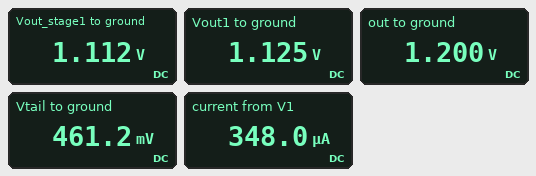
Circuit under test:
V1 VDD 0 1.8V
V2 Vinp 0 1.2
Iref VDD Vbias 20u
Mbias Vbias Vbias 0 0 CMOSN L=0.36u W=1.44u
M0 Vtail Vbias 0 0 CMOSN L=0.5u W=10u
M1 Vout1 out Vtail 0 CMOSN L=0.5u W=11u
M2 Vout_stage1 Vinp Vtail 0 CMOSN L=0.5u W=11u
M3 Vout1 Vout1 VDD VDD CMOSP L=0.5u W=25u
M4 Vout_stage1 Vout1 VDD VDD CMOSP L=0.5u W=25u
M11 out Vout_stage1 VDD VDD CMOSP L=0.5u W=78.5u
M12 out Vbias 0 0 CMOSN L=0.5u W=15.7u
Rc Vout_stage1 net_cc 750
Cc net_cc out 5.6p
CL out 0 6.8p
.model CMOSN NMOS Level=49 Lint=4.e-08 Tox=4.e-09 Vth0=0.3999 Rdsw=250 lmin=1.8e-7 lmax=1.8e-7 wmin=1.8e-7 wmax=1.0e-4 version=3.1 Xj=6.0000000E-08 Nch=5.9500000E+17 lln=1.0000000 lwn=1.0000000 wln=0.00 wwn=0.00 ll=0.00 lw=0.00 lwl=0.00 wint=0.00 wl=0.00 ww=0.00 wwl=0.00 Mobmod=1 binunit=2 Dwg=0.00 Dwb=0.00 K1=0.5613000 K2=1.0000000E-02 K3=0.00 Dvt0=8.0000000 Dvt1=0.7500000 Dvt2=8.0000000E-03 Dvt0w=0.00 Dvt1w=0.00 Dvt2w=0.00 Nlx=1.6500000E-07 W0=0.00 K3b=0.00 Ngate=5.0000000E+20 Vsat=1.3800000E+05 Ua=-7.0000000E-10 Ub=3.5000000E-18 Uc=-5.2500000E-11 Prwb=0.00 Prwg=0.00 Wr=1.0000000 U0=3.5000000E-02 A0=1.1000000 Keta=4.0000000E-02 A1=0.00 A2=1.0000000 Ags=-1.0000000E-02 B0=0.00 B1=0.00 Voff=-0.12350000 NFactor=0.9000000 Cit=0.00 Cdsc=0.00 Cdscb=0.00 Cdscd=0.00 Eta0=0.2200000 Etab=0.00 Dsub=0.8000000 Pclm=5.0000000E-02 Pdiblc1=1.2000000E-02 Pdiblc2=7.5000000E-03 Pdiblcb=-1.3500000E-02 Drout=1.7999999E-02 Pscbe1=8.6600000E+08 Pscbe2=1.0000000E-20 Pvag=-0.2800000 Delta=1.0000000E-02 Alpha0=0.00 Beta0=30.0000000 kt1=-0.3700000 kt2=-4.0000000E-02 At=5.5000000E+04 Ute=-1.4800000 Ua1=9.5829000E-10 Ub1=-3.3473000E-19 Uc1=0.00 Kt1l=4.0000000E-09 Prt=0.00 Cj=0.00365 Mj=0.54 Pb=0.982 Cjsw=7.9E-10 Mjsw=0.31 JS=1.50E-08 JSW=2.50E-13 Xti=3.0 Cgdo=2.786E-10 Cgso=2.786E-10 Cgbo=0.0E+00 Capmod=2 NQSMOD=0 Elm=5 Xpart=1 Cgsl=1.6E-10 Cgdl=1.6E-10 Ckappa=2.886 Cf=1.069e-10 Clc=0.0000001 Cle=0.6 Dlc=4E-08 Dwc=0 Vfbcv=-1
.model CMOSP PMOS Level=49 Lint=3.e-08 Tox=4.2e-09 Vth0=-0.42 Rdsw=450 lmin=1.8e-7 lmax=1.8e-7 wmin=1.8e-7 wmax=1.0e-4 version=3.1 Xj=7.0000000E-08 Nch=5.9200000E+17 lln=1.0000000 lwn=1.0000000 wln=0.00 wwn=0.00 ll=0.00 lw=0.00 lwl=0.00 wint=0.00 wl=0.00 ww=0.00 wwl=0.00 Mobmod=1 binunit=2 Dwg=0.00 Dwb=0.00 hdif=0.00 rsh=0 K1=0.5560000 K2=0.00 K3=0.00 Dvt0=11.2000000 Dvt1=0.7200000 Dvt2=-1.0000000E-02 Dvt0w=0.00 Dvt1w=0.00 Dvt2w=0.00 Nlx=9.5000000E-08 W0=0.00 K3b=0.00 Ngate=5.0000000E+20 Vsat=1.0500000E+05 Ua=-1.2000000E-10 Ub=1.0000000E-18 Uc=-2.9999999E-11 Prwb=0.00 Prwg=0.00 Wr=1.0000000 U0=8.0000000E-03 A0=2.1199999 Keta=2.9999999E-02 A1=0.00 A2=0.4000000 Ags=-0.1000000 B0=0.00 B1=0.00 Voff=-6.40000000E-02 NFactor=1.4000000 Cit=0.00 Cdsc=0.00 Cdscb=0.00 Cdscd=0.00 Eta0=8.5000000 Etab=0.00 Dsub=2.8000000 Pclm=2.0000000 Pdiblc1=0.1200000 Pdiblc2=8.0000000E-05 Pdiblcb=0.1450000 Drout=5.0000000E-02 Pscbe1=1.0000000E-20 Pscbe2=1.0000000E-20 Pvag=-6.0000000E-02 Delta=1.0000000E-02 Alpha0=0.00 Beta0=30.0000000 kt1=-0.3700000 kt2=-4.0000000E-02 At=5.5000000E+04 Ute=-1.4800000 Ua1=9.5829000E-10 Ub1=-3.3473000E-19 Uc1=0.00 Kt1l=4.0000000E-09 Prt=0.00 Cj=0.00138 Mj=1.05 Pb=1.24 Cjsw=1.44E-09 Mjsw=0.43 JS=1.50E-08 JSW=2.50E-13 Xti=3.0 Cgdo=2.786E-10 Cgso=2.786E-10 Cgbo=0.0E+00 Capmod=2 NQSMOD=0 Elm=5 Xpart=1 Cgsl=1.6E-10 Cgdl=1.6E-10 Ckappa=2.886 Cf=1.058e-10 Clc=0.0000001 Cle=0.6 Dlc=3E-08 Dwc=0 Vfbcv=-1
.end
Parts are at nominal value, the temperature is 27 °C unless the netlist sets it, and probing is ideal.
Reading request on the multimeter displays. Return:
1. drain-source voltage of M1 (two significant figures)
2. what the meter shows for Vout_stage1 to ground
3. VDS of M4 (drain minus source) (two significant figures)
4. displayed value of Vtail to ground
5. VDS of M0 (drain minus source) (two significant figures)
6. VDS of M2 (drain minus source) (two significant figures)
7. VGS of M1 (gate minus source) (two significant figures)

660 mV
1.112 V
-690 mV
461.2 mV
460 mV
650 mV
740 mV
